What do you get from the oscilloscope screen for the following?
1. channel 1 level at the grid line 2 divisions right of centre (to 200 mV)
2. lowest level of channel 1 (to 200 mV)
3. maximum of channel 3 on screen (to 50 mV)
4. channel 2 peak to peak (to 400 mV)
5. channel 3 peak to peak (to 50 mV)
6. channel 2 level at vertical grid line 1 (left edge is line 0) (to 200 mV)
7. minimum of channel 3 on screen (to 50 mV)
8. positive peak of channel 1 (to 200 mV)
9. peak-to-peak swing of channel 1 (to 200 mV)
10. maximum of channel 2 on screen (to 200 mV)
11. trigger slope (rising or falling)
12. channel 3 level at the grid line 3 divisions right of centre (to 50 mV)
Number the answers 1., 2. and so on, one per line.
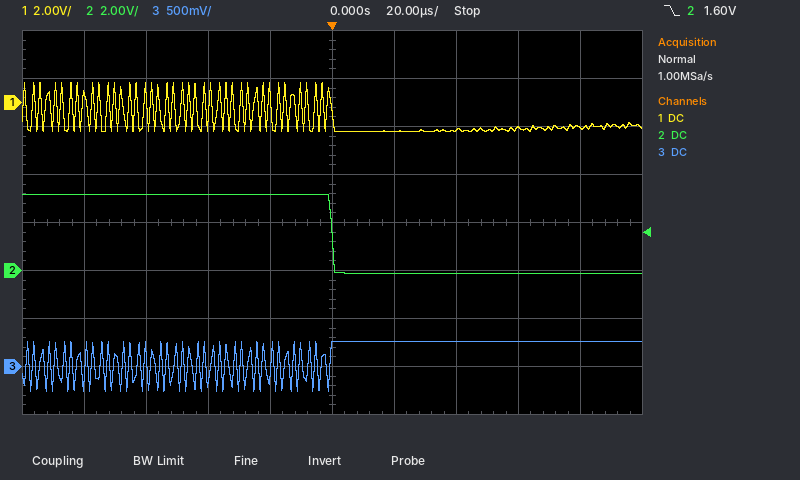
1. -1.2 V
2. -1.2 V
3. 250 mV
4. 3.2 V
5. 500 mV
6. 3.2 V
7. -250 mV
8. 800 mV
9. 2.0 V
10. 3.2 V
11. falling
12. 250 mV
